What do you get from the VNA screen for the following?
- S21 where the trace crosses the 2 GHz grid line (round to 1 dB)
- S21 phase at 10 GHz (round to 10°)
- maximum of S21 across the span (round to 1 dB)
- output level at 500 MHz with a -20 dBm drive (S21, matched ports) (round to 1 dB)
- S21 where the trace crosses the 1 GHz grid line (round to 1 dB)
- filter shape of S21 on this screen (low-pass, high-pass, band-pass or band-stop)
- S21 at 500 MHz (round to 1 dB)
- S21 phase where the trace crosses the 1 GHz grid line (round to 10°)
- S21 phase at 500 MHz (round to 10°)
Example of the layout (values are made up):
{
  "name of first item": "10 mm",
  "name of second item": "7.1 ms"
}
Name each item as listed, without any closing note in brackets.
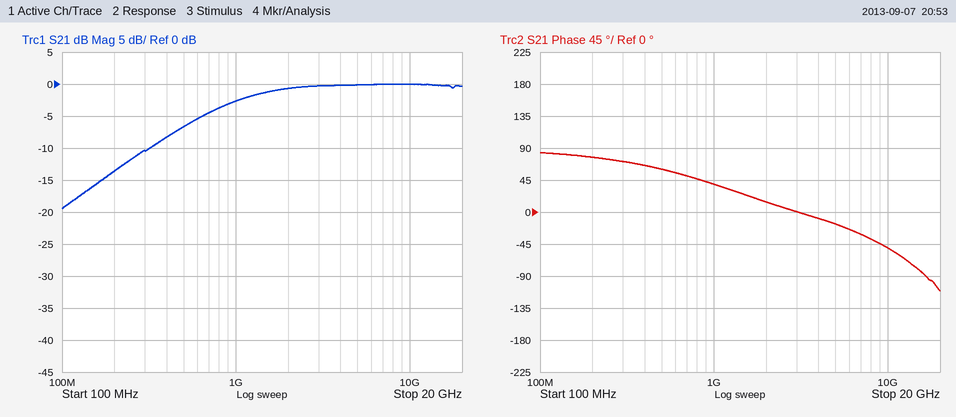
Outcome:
{
  "S21 where the trace crosses the 2 GHz grid line": "-1 dB",
  "S21 phase at 10 GHz": "-50°",
  "maximum of S21 across the span": "0 dB",
  "output level at 500 MHz with a -20 dBm drive (S21, matched ports)": "-27 dBm",
  "S21 where the trace crosses the 1 GHz grid line": "-3 dB",
  "filter shape of S21 on this screen": "high-pass",
  "S21 at 500 MHz": "-7 dB",
  "S21 phase where the trace crosses the 1 GHz grid line": "40°",
  "S21 phase at 500 MHz": "60°"
}
